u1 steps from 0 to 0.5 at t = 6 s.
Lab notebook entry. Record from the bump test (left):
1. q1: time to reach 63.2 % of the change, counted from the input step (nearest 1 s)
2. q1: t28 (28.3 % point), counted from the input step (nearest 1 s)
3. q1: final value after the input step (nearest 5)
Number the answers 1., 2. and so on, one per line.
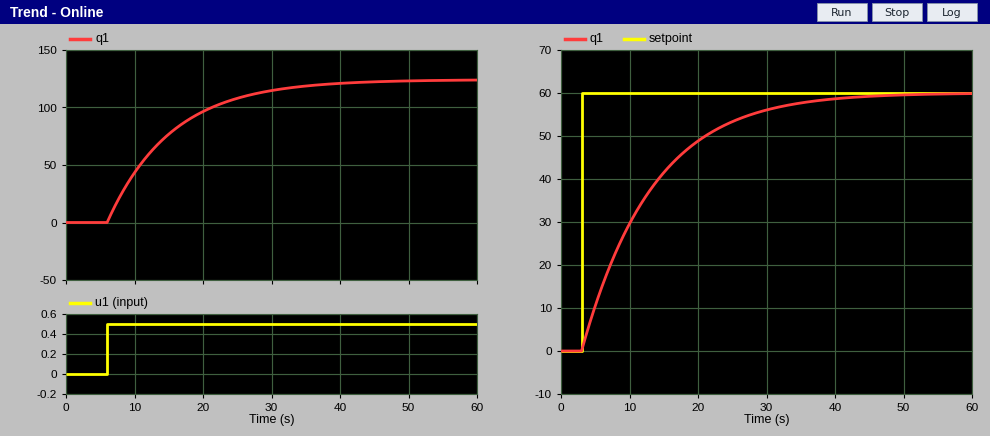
1. 9 s
2. 3 s
3. 125
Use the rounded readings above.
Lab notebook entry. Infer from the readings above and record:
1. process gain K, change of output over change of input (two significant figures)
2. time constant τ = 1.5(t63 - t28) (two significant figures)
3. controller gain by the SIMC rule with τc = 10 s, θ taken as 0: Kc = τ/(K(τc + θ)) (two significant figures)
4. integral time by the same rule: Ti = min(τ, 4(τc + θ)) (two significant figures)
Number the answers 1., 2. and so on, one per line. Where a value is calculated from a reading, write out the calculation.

1. (125 - 0) / 0.5 = 250
2. 1.5 × (9 - 3) = 9.0 s
3. 9 / (250 × (10 + 0)) = 0.0036
4. min(9, 4 × (10 + 0)) = 9.0 s
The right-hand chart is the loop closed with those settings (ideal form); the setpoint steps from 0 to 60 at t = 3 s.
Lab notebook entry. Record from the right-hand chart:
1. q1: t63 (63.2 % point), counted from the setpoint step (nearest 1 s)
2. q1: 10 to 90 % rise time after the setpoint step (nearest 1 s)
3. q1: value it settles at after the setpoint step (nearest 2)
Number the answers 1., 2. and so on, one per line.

1. 10 s
2. 22 s
3. 60
